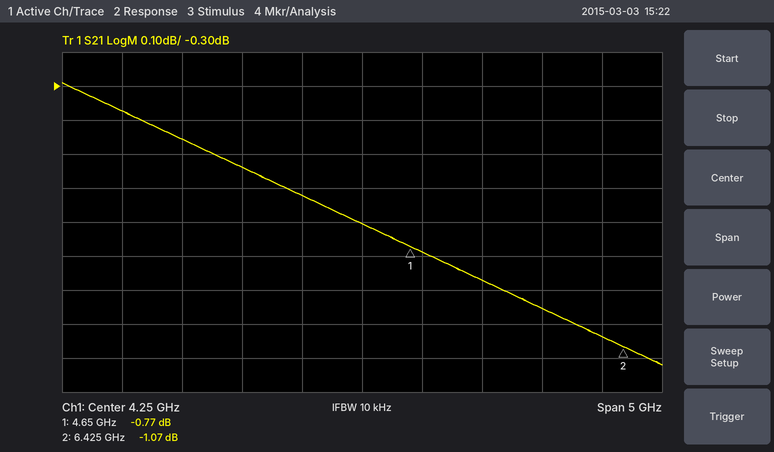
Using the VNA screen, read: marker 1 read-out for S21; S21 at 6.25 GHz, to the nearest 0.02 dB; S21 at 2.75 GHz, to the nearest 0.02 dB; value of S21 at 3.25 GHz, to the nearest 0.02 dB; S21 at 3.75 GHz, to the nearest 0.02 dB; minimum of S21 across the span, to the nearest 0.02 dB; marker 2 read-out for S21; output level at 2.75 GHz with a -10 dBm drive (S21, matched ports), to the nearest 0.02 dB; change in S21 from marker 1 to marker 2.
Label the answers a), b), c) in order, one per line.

a) -0.77 dB
b) -1.04 dB
c) -0.46 dB
d) -0.54 dB
e) -0.62 dB
f) -1.12 dB
g) -1.07 dB
h) -10.46 dBm
i) -0.30 dB
